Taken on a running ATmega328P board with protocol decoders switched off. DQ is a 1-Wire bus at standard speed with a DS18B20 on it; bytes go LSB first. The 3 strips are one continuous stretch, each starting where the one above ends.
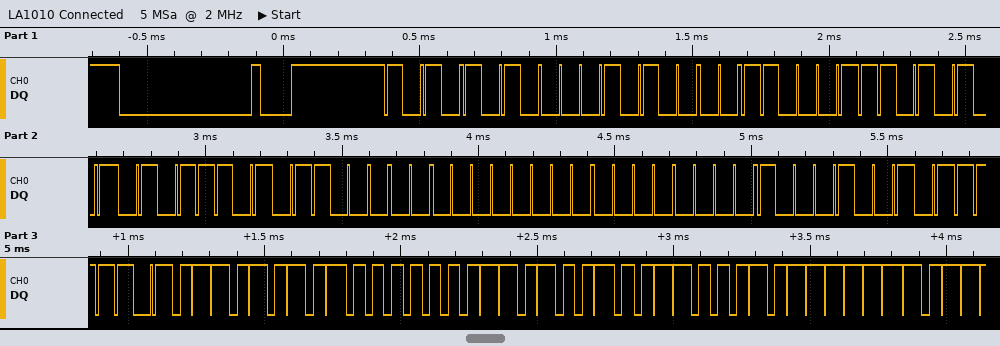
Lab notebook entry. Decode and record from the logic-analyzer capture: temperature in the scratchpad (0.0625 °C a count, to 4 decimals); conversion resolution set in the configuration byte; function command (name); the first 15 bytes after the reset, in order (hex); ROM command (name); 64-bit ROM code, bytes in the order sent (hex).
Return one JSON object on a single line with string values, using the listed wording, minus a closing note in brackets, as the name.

{"temperature in the scratchpad": "21.3750 °C", "conversion resolution set in the configuration byte": "12 bits", "function command": "Read Scratchpad", "the first 15 bytes after the reset, in order": "55 28 8C AB BA 06 00 00 91 BE 56 01 4B 46 7F", "ROM command": "Match ROM", "64-bit ROM code, bytes in the order sent": "28 8C AB BA 06 00 00 91"}
